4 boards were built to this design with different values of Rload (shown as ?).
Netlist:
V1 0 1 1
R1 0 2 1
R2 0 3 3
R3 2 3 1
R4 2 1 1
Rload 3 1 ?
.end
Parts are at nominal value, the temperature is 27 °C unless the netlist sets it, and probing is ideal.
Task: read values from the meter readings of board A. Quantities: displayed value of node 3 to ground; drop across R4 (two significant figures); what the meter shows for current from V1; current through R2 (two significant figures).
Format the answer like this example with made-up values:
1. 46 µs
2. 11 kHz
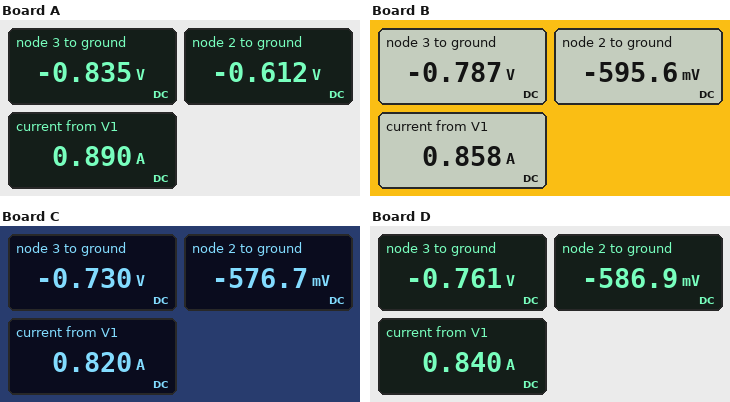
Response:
1. -0.835 V
2. 390 mV
3. 0.890 A
4. 280 mA
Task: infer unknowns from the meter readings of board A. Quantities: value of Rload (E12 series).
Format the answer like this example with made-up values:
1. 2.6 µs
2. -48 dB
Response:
1. 0.33 Ω
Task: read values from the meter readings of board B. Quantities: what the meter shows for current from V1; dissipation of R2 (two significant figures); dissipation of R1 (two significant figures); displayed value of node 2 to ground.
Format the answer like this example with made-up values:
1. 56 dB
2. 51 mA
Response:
1. 0.858 A
2. 210 mW
3. 350 mW
4. -595.6 mV
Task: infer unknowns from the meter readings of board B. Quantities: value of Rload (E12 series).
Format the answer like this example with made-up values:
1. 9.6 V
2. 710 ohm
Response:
1. 0.47 Ω
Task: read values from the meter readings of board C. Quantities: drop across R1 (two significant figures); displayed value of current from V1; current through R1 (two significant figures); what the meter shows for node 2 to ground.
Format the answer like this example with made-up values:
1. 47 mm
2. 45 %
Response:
1. 580 mV
2. 0.820 A
3. 580 mA
4. -576.7 mV
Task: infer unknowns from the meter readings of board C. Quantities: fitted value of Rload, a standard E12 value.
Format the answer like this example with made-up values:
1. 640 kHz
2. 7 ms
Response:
1. 0.68 Ω
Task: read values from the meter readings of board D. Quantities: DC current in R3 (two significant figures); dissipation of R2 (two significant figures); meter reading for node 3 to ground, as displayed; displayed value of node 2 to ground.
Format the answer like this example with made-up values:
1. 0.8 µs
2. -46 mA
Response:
1. 170 mA
2. 190 mW
3. -0.761 V
4. -586.9 mV
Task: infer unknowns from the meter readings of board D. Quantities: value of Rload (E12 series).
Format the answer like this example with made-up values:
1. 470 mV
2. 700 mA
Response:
1. 0.56 Ω
